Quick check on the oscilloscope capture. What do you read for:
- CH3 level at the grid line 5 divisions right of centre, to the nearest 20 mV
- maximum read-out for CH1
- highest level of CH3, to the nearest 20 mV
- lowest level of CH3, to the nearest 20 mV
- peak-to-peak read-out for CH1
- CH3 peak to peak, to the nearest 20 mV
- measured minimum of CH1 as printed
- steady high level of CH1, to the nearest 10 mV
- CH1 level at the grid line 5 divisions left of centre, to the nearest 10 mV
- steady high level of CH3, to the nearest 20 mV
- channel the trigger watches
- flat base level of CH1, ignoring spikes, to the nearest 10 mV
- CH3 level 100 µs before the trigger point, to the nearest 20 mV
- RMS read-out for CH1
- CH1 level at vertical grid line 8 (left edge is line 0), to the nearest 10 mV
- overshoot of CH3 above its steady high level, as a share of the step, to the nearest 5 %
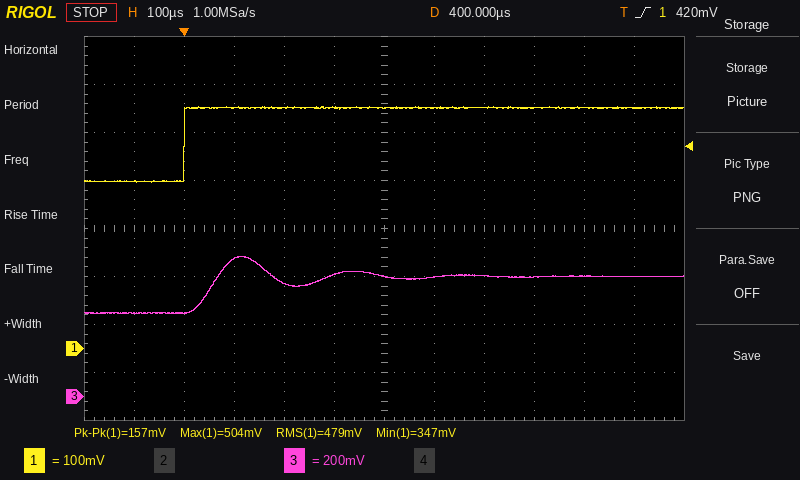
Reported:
500 mV
504 mV
580 mV
340 mV
157 mV
240 mV
347 mV
500 mV
350 mV
500 mV
CH1
350 mV
340 mV
479 mV
500 mV
55 %
